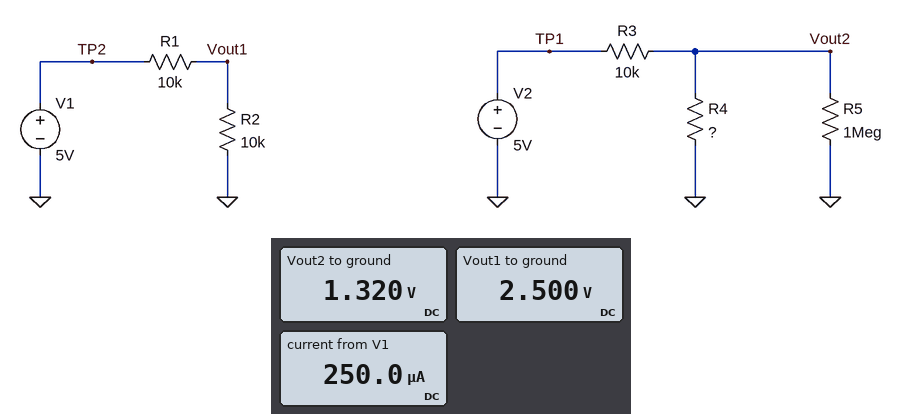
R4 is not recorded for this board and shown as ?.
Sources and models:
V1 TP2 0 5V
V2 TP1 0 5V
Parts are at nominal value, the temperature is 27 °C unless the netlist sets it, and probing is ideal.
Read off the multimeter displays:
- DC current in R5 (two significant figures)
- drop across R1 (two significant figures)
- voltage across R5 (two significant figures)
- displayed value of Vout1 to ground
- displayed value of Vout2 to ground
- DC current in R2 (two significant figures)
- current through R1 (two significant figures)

1.3 µA
2.5 V
1.3 V
2.500 V
1.320 V
250 µA
250 µA
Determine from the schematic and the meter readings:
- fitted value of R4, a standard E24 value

3.6 kΩ
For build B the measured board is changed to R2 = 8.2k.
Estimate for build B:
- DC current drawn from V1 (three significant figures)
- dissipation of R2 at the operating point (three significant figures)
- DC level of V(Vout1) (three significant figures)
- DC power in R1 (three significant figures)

275 µA
619 µW
2.25 V
755 µW
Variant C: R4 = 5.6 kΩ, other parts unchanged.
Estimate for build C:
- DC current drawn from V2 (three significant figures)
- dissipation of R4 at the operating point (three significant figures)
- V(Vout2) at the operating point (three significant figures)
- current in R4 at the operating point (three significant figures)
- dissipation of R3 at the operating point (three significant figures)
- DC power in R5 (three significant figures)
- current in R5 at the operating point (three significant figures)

321 µA
571 µW
1.79 V
319 µA
1.03 mW
3.20 µW
1.79 µA
